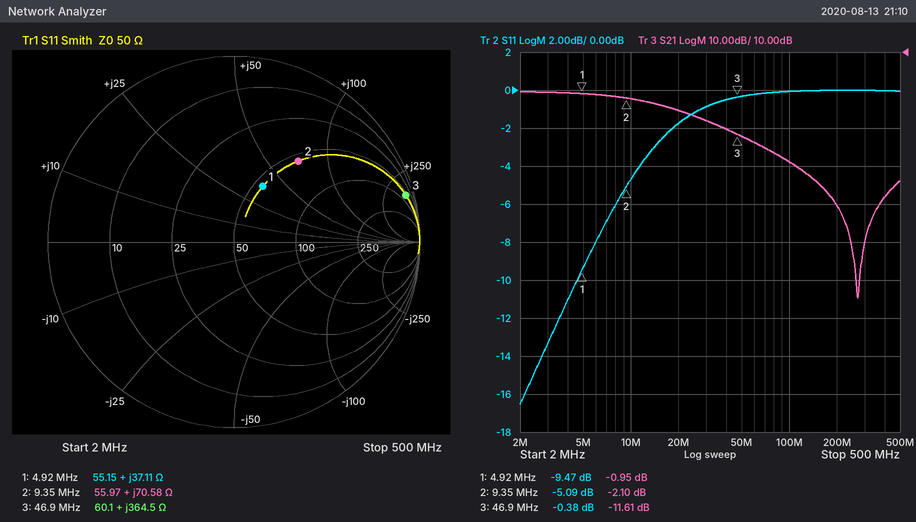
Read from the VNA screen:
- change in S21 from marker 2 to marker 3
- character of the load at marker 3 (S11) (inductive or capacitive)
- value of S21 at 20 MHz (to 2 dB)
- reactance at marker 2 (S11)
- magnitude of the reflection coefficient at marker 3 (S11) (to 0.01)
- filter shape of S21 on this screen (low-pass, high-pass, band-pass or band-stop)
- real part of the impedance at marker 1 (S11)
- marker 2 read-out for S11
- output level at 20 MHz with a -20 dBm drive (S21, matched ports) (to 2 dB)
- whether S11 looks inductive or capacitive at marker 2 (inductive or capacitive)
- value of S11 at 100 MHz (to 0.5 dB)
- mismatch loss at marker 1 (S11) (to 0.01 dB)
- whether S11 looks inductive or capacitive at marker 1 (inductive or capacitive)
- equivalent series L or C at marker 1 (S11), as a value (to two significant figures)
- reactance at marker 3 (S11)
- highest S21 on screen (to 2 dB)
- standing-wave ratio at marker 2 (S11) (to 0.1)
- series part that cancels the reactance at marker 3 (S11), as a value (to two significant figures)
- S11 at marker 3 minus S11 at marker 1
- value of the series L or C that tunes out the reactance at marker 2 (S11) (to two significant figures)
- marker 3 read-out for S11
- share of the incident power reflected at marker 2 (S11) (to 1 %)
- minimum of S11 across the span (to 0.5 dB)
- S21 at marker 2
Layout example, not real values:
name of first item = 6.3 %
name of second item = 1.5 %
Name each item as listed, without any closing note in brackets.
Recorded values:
change in S21 from marker 2 to marker 3 = -9.51 dB
character of the load at marker 3 (S11) = inductive
value of S21 at 20 MHz = -6 dB
reactance at marker 2 = +70.58 Ω
magnitude of the reflection coefficient at marker 3 (S11) = 0.96
filter shape of S21 on this screen = low-pass
real part of the impedance at marker 1 = 55.15 Ω
marker 2 read-out for S11 = -5.09 dB
output level at 20 MHz with a -20 dBm drive (S21, matched ports) = -26 dBm
whether S11 looks inductive or capacitive at marker 2 = inductive
value of S11 at 100 MHz = 0.0 dB
mismatch loss at marker 1 (S11) = 0.52 dB
whether S11 looks inductive or capacitive at marker 1 = inductive
equivalent series L or C at marker 1 (S11), as a value = 1.2 µH
reactance at marker 3 = +364.5 Ω
highest S21 on screen = 0 dB
standing-wave ratio at marker 2 (S11) = 3.5
series part that cancels the reactance at marker 3 (S11), as a value = 9.3 pF
S11 at marker 3 minus S11 at marker 1 = 9.09 dB
value of the series L or C that tunes out the reactance at marker 2 (S11) = 240 pF
marker 3 read-out for S11 = -0.38 dB
share of the incident power reflected at marker 2 (S11) = 31 %
minimum of S11 across the span = -16.5 dB
S21 at marker 2 = -2.10 dB
